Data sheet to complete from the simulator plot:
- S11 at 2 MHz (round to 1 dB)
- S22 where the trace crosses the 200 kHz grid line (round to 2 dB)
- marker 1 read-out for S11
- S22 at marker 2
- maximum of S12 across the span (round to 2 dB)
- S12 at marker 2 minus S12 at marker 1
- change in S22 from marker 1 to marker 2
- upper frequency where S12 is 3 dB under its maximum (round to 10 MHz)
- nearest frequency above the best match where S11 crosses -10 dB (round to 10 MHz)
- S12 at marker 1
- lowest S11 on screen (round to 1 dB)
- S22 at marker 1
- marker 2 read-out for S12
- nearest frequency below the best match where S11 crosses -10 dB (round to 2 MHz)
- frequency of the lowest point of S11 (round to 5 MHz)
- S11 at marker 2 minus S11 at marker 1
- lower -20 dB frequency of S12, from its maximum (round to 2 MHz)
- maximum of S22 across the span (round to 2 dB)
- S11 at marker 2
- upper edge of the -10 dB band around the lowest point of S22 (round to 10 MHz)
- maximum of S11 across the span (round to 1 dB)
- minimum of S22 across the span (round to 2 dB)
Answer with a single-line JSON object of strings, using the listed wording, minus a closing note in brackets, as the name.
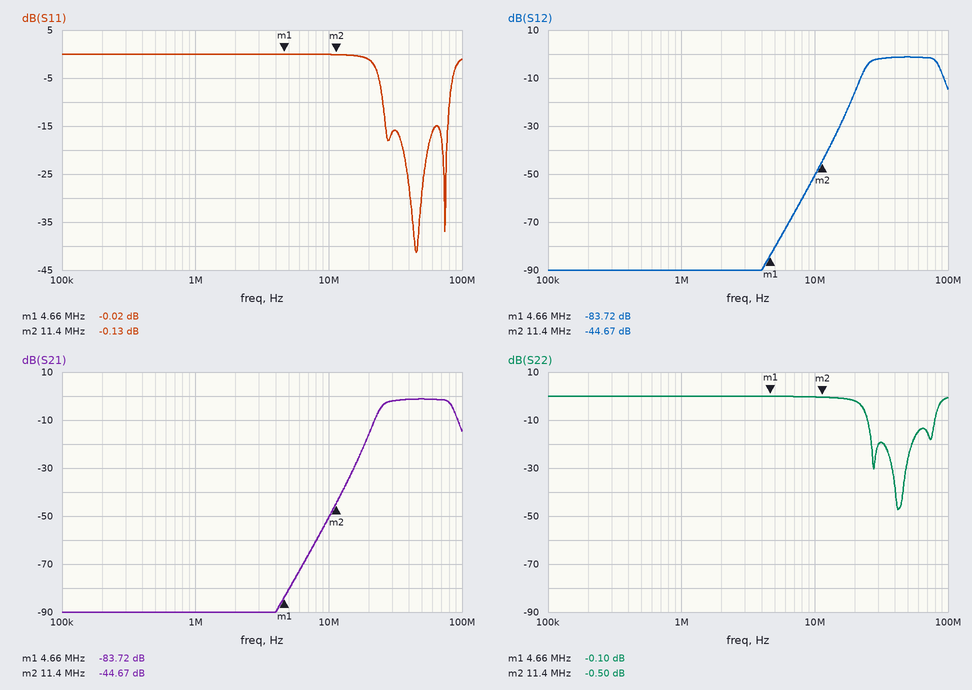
{"S11 at 2 MHz": "0 dB", "S22 where the trace crosses the 200 kHz grid line": "0 dB", "marker 1 read-out for S11": "-0.02 dB", "S22 at marker 2": "-0.50 dB", "maximum of S12 across the span": "-2 dB", "S12 at marker 2 minus S12 at marker 1": "39.05 dB", "change in S22 from marker 1 to marker 2": "-0.40 dB", "upper frequency where S12 is 3 dB under its maximum": "80 MHz", "nearest frequency above the best match where S11 crosses -10 dB": "80 MHz", "S12 at marker 1": "-83.72 dB", "lowest S11 on screen": "-41 dB", "S22 at marker 1": "-0.10 dB", "marker 2 read-out for S12": "-44.67 dB", "nearest frequency below the best match where S11 crosses -10 dB": "26 MHz", "frequency of the lowest point of S11": "45 MHz", "S11 at marker 2 minus S11 at marker 1": "-0.11 dB", "lower -20 dB frequency of S12, from its maximum": "18 MHz", "maximum of S22 across the span": "0 dB", "S11 at marker 2": "-0.13 dB", "upper edge of the -10 dB band around the lowest point of S22": "80 MHz", "maximum of S11 across the span": "0 dB", "minimum of S22 across the span": "-48 dB"}
